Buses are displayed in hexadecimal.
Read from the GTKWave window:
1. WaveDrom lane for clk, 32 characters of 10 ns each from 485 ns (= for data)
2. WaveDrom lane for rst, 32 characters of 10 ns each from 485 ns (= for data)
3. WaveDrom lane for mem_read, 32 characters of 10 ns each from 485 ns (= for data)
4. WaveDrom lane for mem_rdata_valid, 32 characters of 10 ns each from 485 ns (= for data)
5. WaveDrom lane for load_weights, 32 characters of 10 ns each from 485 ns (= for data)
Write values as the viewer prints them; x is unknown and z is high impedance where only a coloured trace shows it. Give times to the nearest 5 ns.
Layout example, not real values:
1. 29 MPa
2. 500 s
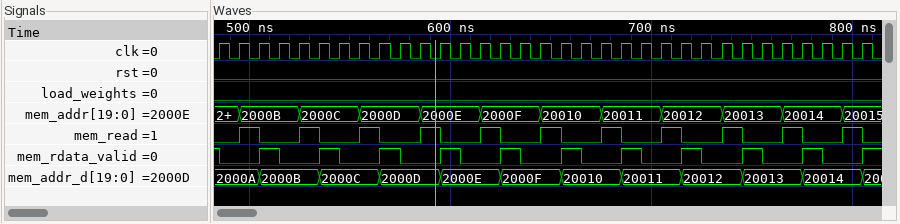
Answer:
1. {name: 'clk', wave: 'p...............................'}
2. {name: 'rst', wave: '0...............................'}
3. {name: 'mem_read', wave: '010.10.10.10.10.10.10.10.10.10.1'}
4. {name: 'mem_rdata_valid', wave: '0.10.10.10.10.10.10.10.10.10.10.'}
5. {name: 'load_weights', wave: '0...............................'}
